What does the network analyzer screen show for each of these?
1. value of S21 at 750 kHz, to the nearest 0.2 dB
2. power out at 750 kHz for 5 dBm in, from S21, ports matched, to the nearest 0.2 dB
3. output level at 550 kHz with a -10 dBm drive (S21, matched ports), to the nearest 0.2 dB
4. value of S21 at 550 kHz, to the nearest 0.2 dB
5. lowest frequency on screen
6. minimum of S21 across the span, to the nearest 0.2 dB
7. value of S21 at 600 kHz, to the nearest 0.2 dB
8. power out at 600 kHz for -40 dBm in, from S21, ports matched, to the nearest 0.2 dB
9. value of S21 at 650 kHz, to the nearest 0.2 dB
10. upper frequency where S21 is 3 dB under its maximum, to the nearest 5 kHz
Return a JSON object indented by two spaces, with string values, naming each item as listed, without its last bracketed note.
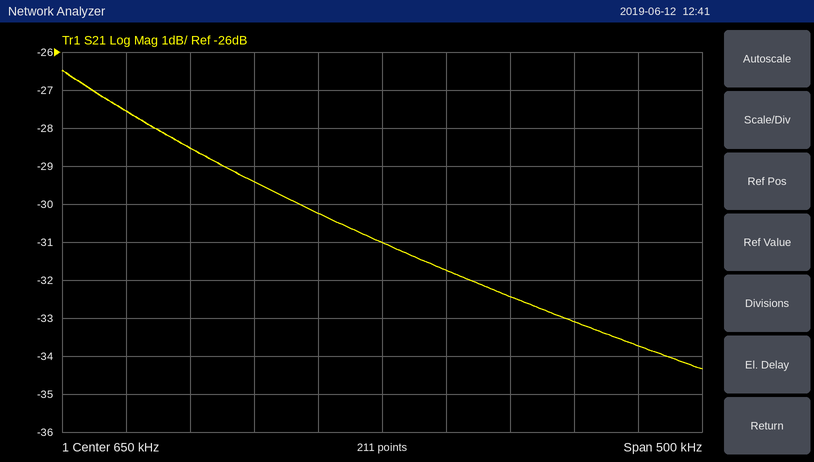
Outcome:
{
  "value of S21 at 750 kHz, to the nearest 0.2 dB": "-32.4 dB",
  "power out at 750 kHz for 5 dBm in, from S21, ports matched, to the nearest 0.2 dB": "-27.4 dBm",
  "output level at 550 kHz with a -10 dBm drive (S21, matched ports), to the nearest 0.2 dB": "-39.4 dBm",
  "value of S21 at 550 kHz, to the nearest 0.2 dB": "-29.4 dB",
  "lowest frequency on screen": "400 kHz",
  "minimum of S21 across the span, to the nearest 0.2 dB": "-34.4 dB",
  "value of S21 at 600 kHz, to the nearest 0.2 dB": "-30.2 dB",
  "power out at 600 kHz for -40 dBm in, from S21, ports matched, to the nearest 0.2 dB": "-70.2 dBm",
  "value of S21 at 650 kHz, to the nearest 0.2 dB": "-31.0 dB",
  "upper frequency where S21 is 3 dB under its maximum, to the nearest 5 kHz": "555 kHz"
}
